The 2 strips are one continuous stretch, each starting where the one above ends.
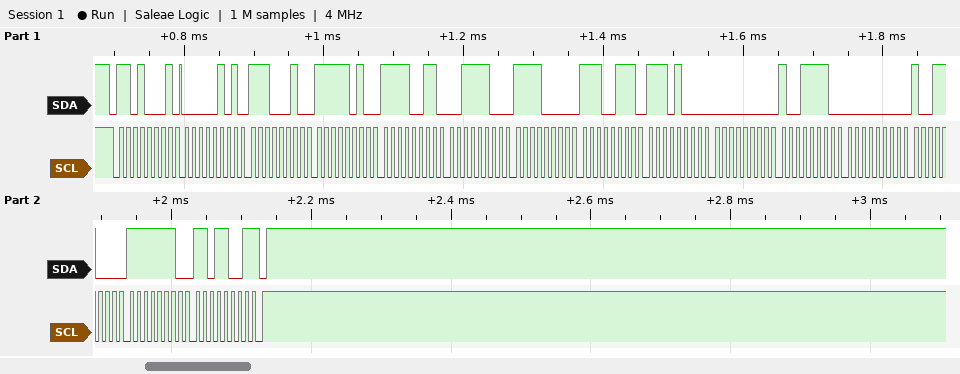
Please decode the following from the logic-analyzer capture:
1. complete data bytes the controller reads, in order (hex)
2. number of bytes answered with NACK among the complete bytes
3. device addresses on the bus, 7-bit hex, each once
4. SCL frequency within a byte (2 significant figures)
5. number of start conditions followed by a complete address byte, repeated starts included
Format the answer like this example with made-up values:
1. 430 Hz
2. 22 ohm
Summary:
1. 05 E2 FA F3 3C F0 E7 E8 00 9E 00 98 FE D9
2. 1
3. 0x68
4. 100 kHz
5. 1
